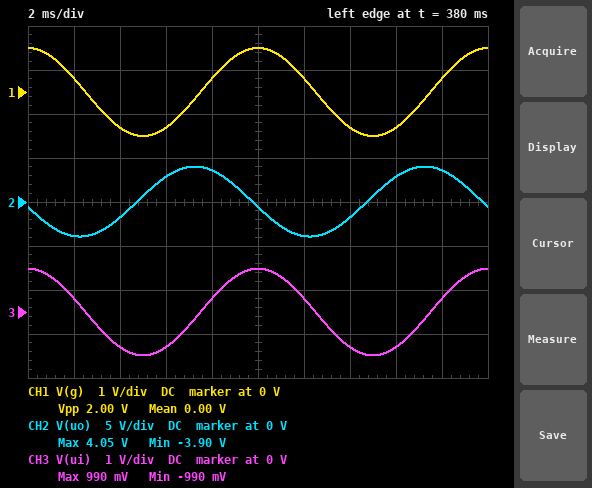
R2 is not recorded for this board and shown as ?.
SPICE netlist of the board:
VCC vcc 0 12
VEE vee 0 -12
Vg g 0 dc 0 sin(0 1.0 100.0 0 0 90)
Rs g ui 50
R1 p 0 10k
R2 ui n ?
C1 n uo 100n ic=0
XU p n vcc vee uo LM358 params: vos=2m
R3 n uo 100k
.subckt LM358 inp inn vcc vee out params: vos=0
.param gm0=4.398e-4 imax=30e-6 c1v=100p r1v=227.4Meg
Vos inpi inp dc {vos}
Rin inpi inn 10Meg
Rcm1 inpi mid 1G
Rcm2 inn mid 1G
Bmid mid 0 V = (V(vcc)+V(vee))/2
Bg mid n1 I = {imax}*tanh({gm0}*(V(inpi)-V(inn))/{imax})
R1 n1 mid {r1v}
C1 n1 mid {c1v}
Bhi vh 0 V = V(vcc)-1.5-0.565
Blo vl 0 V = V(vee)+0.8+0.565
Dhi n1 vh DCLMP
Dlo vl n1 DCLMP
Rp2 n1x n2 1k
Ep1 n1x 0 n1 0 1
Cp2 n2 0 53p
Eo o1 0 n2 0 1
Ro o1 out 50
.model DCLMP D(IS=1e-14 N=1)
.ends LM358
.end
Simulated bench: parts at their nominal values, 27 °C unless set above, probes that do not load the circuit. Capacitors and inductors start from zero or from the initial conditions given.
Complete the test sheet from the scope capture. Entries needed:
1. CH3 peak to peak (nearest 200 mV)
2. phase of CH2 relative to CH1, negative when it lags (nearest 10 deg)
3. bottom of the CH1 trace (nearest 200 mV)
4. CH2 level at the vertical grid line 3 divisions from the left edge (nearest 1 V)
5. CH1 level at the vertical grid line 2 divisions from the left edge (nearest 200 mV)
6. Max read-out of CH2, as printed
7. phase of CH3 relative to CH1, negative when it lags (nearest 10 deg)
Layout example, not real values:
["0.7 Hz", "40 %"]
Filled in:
["2.0 V", "100 deg", "-1.0 V", "3 V", "-800 mV", "4.05 V", "0 deg"]
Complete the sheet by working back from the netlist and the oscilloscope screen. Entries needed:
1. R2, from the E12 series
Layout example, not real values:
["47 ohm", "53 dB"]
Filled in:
["3.9 kΩ"]
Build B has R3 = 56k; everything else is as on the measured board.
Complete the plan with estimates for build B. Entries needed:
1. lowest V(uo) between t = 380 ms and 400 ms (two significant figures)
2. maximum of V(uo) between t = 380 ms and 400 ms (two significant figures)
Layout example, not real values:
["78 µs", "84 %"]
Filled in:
["-3.8 V", "3.9 V"]
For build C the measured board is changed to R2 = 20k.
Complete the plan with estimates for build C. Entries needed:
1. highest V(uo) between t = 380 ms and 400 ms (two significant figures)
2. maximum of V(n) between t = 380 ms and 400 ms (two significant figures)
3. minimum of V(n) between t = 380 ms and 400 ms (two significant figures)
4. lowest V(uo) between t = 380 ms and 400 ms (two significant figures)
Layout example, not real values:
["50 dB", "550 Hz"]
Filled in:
["800 mV", "2.1 mV", "1.9 mV", "-770 mV"]
